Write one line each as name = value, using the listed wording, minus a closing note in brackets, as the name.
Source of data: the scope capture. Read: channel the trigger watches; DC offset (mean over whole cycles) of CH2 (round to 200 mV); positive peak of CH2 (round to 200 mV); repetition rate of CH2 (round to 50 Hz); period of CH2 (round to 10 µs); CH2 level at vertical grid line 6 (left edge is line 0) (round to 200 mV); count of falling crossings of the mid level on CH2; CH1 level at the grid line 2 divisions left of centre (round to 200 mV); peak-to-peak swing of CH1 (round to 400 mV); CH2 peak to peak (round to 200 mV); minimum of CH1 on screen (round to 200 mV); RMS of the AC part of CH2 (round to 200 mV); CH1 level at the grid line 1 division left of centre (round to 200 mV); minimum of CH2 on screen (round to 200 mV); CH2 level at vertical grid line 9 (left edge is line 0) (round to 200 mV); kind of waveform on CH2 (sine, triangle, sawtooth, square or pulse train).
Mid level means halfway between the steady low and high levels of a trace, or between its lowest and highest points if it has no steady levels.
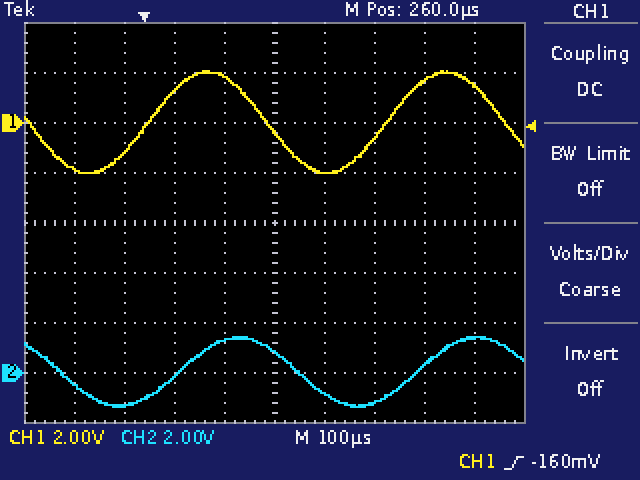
channel the trigger watches = CH1
DC offset (mean over whole cycles) of CH2 = 0.0 V
positive peak of CH2 = 1.4 V
repetition rate of CH2 = 2.10 kHz
period of CH2 = 480 µs
CH2 level at vertical grid line 6 (left edge is line 0) = -800 mV
count of falling crossings of the mid level on CH2 = 2
CH1 level at the grid line 2 divisions left of centre = 1.2 V
peak-to-peak swing of CH1 = 4.0 V
CH2 peak to peak = 2.8 V
minimum of CH1 on screen = -2.0 V
RMS of the AC part of CH2 = 1.0 V
CH1 level at the grid line 1 division left of centre = 1.8 V
minimum of CH2 on screen = -1.4 V
CH2 level at vertical grid line 9 (left edge is line 0) = 1.4 V
kind of waveform on CH2 = sine
